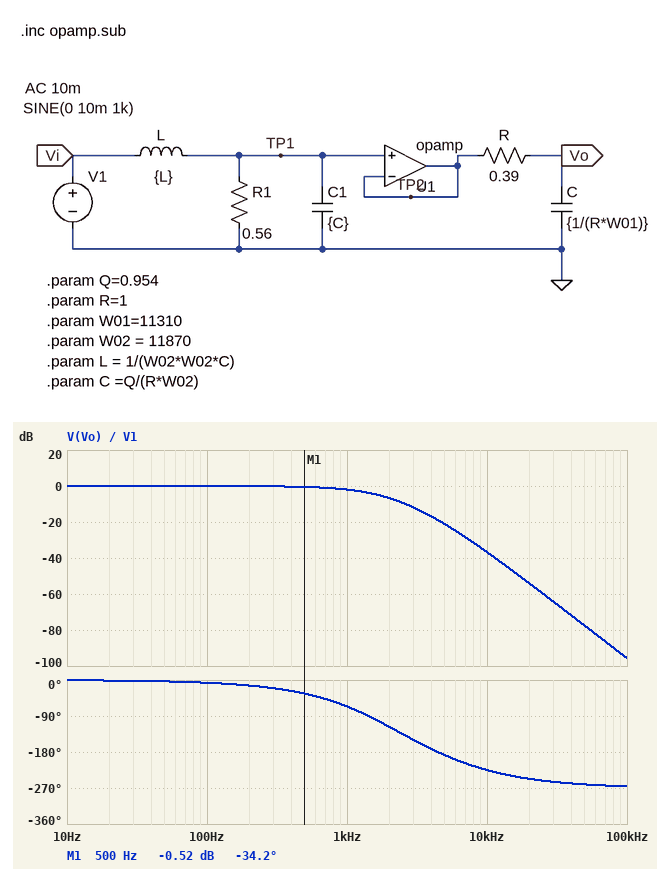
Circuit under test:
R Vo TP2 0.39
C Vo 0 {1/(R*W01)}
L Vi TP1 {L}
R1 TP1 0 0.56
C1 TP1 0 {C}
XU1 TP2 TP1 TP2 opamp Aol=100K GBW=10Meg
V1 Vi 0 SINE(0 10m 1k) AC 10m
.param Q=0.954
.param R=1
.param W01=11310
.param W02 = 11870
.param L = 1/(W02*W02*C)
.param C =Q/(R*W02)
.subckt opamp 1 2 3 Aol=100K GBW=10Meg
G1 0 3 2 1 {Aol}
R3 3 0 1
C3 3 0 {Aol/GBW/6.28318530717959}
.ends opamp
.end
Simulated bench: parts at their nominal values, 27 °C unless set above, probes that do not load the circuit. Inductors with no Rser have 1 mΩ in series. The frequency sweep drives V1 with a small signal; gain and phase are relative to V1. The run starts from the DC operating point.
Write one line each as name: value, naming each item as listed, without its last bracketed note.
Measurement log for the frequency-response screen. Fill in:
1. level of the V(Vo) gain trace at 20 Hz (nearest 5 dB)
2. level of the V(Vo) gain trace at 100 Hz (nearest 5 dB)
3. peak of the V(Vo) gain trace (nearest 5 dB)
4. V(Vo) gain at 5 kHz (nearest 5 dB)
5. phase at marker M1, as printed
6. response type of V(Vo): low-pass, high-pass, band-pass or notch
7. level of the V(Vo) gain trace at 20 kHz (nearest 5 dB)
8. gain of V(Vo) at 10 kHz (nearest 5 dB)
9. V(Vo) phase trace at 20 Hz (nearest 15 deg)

level of the V(Vo) gain trace at 20 Hz: 0 dB
level of the V(Vo) gain trace at 100 Hz: 0 dB
peak of the V(Vo) gain trace: 0 dB
V(Vo) gain at 5 kHz: -20 dB
phase at marker M1, as printed: -34.2 deg
response type of V(Vo): low-pass, high-pass, band-pass or notch: low-pass
level of the V(Vo) gain trace at 20 kHz: -55 dB
gain of V(Vo) at 10 kHz: -35 dB
V(Vo) phase trace at 20 Hz: 0 deg
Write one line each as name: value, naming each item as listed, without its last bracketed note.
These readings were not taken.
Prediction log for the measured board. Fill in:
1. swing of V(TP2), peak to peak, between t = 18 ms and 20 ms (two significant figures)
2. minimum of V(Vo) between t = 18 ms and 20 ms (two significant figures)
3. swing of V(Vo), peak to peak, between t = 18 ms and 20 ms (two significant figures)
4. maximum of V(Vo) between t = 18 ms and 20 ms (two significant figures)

swing of V(TP2), peak to peak, between t = 18 ms and 20 ms: 16 mV
minimum of V(Vo) between t = 18 ms and 20 ms: -8.0 mV
swing of V(Vo), peak to peak, between t = 18 ms and 20 ms: 16 mV
maximum of V(Vo) between t = 18 ms and 20 ms: 8.0 mV
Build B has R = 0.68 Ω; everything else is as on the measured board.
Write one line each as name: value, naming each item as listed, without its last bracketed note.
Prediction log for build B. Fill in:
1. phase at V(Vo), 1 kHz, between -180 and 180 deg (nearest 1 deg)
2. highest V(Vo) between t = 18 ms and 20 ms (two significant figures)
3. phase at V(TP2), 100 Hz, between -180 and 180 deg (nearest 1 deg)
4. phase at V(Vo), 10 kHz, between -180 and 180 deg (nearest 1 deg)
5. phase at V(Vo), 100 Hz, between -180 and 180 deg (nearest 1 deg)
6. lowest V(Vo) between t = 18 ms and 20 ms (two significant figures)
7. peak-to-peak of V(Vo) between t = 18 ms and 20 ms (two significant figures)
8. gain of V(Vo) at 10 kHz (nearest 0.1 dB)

phase at V(Vo), 1 kHz, between -180 and 180 deg: -75 deg
highest V(Vo) between t = 18 ms and 20 ms: 7.6 mV
phase at V(TP2), 100 Hz, between -180 and 180 deg: -6 deg
phase at V(Vo), 10 kHz, between -180 and 180 deg: 125 deg
phase at V(Vo), 100 Hz, between -180 and 180 deg: -8 deg
lowest V(Vo) between t = 18 ms and 20 ms: -7.6 mV
peak-to-peak of V(Vo) between t = 18 ms and 20 ms: 15 mV
gain of V(Vo) at 10 kHz: -41.0 dB
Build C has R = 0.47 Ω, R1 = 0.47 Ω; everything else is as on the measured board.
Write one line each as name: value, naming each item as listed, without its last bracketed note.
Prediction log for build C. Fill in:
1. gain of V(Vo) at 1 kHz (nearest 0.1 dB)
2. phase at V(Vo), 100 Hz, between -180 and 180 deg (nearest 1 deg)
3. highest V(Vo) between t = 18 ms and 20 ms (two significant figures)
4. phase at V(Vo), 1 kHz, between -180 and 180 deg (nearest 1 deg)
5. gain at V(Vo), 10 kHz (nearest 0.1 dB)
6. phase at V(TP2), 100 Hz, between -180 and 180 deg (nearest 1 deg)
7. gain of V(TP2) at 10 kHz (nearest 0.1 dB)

gain of V(Vo) at 1 kHz: -3.1 dB
phase at V(Vo), 100 Hz, between -180 and 180 deg: -8 deg
highest V(Vo) between t = 18 ms and 20 ms: 7.0 mV
phase at V(Vo), 1 kHz, between -180 and 180 deg: -73 deg
gain at V(Vo), 10 kHz: -38.3 dB
phase at V(TP2), 100 Hz, between -180 and 180 deg: -7 deg
gain of V(TP2) at 10 kHz: -29.4 dB
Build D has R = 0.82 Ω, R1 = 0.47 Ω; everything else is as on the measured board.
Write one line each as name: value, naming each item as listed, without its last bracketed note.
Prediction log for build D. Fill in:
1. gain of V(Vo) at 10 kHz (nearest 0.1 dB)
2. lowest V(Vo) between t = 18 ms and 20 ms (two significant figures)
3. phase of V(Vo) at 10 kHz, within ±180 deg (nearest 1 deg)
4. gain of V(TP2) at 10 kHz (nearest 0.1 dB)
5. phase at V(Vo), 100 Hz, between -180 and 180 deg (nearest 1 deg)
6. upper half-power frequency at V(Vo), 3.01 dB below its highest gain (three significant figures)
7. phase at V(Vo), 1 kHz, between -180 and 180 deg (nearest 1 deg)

gain of V(Vo) at 10 kHz: -42.8 dB
lowest V(Vo) between t = 18 ms and 20 ms: -6.6 mV
phase of V(Vo) at 10 kHz, within ±180 deg: 126 deg
gain of V(TP2) at 10 kHz: -29.4 dB
phase at V(Vo), 100 Hz, between -180 and 180 deg: -9 deg
upper half-power frequency at V(Vo), 3.01 dB below its highest gain: 895 Hz
phase at V(Vo), 1 kHz, between -180 and 180 deg: -83 deg
